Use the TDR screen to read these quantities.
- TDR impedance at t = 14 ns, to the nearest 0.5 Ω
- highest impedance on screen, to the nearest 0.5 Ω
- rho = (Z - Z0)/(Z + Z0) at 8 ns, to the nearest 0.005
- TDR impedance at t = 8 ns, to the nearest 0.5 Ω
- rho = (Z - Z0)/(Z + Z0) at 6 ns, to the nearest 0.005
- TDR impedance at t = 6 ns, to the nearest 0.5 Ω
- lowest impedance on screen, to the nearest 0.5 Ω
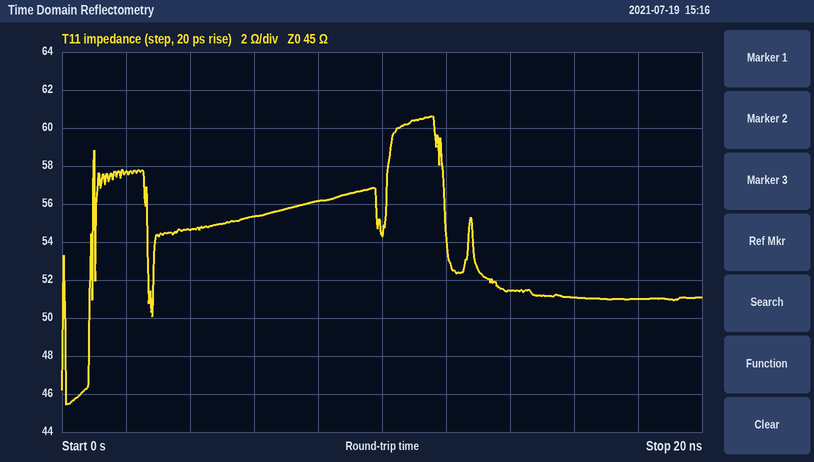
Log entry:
51.5 Ω
60.5 Ω
+0.110
56.0 Ω
+0.105
55.5 Ω
45.5 Ω
